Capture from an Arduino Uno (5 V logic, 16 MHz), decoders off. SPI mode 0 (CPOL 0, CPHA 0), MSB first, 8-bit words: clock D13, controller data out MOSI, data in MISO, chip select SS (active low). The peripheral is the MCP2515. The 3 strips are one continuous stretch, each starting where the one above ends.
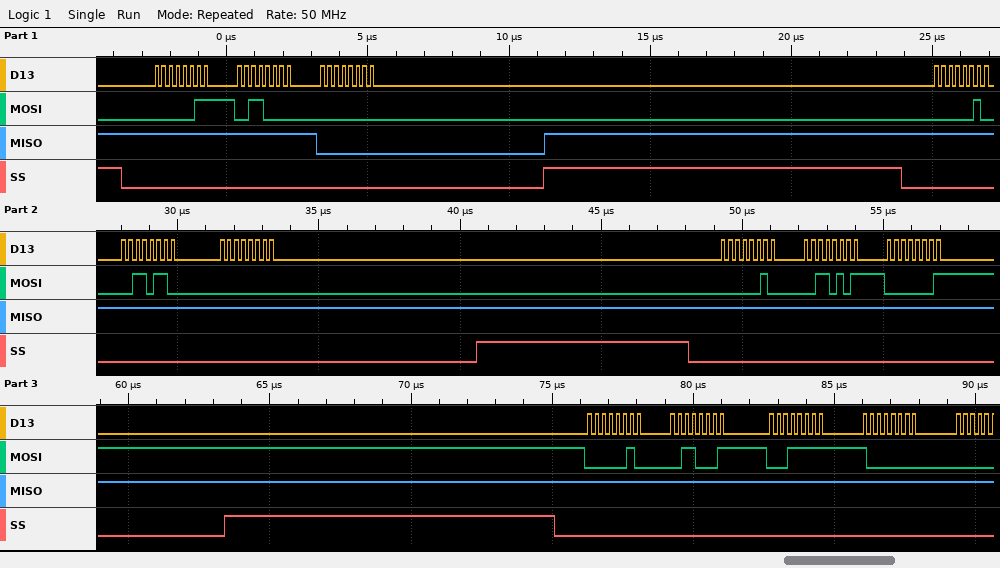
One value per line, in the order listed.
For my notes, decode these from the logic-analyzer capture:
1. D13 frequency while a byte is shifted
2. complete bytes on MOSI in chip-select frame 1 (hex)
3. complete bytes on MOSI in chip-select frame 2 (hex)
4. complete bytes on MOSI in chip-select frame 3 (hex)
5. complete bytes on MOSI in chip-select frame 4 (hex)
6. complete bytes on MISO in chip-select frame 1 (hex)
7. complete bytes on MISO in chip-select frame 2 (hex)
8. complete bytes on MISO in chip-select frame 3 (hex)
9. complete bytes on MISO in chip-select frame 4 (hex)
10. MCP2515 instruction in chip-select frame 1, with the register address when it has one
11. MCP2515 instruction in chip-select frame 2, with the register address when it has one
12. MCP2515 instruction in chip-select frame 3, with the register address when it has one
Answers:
4 MHz
03 30 00
02 36 00
02 35 01
02 31 1F 80
FF FF 00
FF FF FF
FF FF FF
FF FF FF FF
READ 0x30
WRITE 0x36
WRITE 0x35
